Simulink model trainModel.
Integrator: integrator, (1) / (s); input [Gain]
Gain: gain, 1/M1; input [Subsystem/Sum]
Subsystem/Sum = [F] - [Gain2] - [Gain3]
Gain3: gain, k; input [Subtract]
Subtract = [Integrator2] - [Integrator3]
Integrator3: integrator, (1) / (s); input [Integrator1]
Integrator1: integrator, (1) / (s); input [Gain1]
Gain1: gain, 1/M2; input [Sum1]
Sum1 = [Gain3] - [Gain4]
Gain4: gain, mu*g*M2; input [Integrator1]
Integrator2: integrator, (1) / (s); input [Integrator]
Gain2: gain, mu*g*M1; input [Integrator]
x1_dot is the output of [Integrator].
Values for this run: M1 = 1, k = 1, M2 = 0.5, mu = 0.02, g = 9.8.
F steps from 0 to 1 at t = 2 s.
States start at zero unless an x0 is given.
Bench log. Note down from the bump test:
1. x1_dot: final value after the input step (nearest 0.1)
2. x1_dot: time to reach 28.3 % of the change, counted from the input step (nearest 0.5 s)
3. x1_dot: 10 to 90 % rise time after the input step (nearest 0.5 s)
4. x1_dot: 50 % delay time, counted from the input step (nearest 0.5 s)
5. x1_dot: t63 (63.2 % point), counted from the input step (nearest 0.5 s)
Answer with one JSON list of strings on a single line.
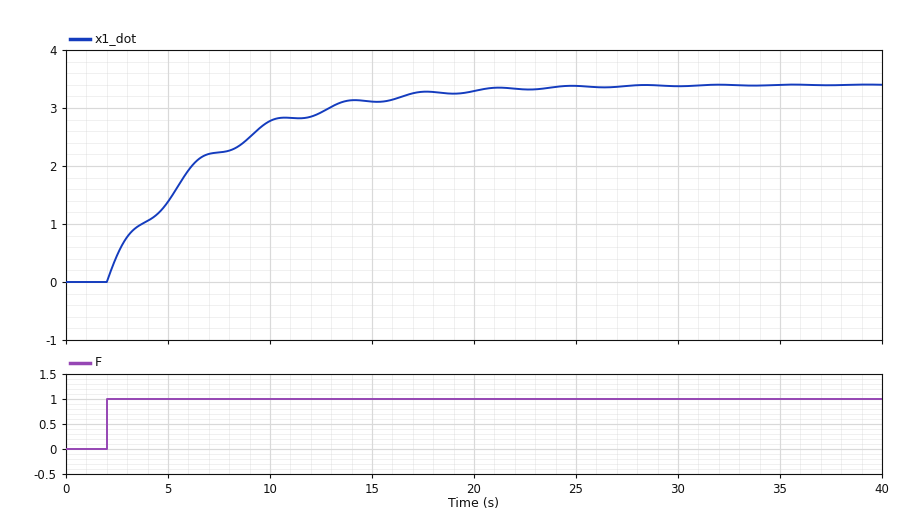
["3.4", "1.5 s", "11.0 s", "3.5 s", "4.5 s"]
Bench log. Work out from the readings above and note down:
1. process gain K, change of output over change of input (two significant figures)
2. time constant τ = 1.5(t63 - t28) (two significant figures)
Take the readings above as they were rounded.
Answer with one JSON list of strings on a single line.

["3.4", "4.5 s"]
